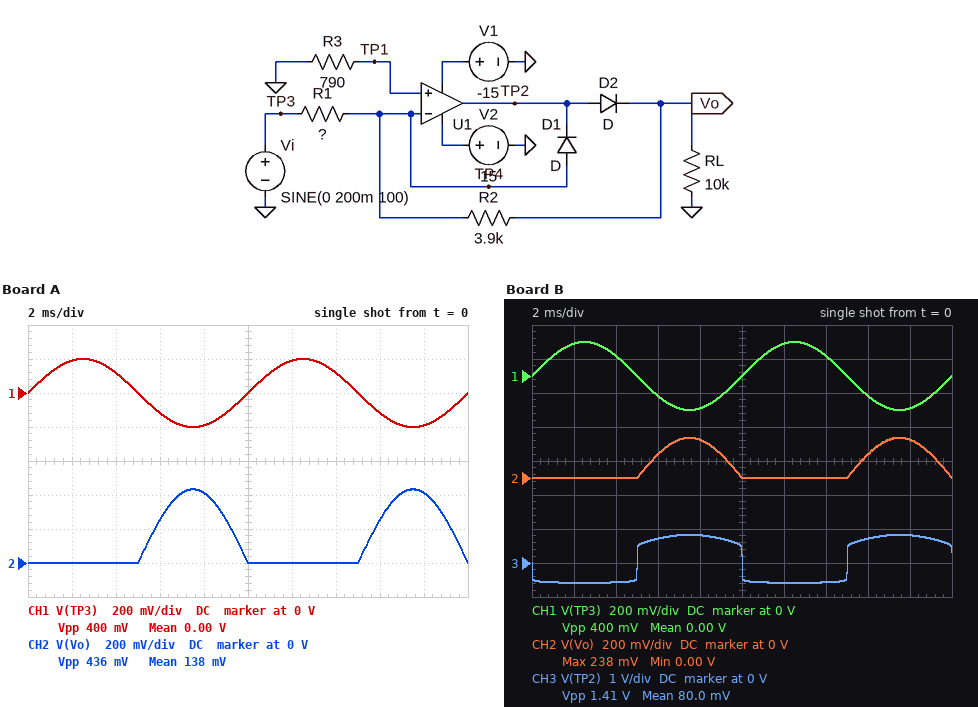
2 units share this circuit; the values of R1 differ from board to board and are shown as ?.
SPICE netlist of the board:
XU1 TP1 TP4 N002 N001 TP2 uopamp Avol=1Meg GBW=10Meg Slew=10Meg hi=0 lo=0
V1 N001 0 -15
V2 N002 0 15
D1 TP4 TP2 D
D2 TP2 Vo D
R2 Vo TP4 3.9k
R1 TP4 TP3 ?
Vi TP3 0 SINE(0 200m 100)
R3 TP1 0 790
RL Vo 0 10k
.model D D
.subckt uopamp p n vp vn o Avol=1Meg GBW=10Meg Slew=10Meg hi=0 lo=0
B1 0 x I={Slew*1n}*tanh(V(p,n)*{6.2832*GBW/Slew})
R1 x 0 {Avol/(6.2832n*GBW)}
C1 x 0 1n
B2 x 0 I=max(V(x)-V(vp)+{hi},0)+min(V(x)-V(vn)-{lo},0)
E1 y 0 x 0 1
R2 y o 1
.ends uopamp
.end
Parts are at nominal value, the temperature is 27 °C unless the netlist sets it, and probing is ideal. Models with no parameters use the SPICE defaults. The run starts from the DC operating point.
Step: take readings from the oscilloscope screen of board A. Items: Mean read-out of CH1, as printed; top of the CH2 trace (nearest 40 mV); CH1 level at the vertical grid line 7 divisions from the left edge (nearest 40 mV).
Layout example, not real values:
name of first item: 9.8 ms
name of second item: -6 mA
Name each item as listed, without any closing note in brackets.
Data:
Mean read-out of CH1, as printed: 0.00 V
top of the CH2 trace: 440 mV
CH1 level at the vertical grid line 7 divisions from the left edge: 120 mV
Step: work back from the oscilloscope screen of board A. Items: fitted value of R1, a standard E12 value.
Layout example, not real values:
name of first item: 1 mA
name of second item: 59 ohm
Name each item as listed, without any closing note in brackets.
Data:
fitted value of R1, a standard E12 value: 1.8 kΩ
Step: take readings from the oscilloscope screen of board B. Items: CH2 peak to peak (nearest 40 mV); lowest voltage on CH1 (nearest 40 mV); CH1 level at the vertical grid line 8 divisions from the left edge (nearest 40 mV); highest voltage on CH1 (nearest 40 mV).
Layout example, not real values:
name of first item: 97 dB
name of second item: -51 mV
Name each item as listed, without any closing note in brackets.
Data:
CH2 peak to peak: 240 mV
lowest voltage on CH1: -200 mV
CH1 level at the vertical grid line 8 divisions from the left edge: -120 mV
highest voltage on CH1: 200 mV
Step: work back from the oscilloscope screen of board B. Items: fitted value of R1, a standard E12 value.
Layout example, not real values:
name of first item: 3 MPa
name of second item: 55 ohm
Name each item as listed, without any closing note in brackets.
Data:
fitted value of R1, a standard E12 value: 3.3 kΩ
